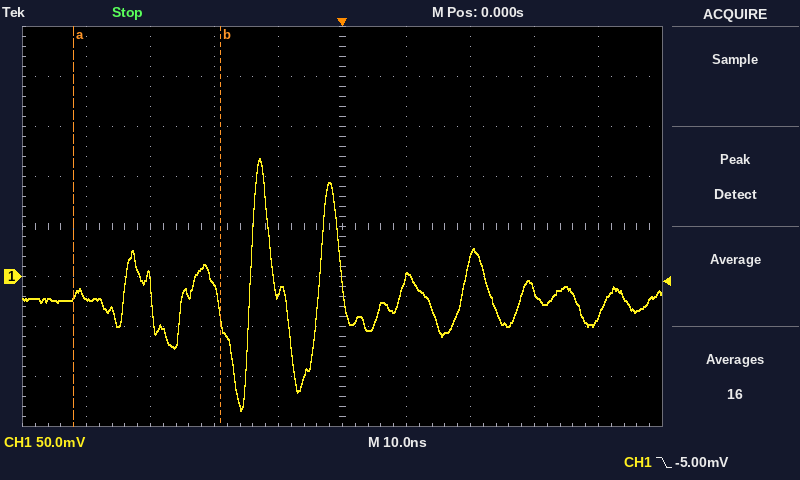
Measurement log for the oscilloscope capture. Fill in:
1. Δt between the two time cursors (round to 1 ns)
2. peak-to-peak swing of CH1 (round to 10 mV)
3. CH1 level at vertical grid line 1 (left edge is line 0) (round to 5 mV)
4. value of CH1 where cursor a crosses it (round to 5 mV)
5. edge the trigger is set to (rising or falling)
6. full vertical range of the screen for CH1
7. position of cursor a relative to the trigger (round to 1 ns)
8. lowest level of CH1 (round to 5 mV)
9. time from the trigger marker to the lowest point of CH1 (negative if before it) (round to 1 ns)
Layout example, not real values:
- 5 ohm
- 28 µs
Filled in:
- 23 ns
- 250 mV
- -20 mV
- -20 mV
- falling
- 400 mV
- -42 ns
- -135 mV
- -16 ns
